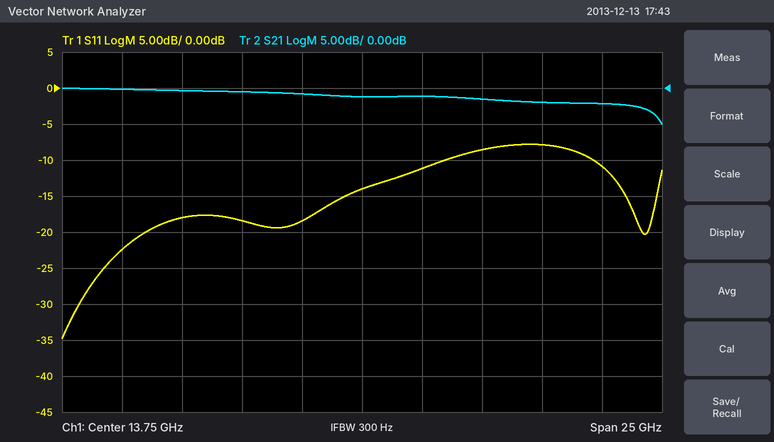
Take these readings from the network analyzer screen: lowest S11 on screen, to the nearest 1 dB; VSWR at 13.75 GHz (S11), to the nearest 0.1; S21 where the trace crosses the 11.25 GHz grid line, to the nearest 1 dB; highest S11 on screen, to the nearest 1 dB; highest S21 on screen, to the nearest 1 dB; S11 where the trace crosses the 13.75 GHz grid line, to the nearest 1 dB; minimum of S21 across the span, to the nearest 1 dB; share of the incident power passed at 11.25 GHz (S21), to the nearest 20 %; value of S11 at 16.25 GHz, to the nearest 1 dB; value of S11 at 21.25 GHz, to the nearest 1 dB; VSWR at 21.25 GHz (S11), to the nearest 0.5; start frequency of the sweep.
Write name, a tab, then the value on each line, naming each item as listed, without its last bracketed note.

lowest S11 on screen, to the nearest 1 dB	-35 dB
VSWR at 13.75 GHz (S11), to the nearest 0.1	1.5
S21 where the trace crosses the 11.25 GHz grid line, to the nearest 1 dB	-1 dB
highest S11 on screen, to the nearest 1 dB	-8 dB
highest S21 on screen, to the nearest 1 dB	0 dB
S11 where the trace crosses the 13.75 GHz grid line, to the nearest 1 dB	-14 dB
minimum of S21 across the span, to the nearest 1 dB	-5 dB
share of the incident power passed at 11.25 GHz (S21), to the nearest 20 %	80 %
value of S11 at 16.25 GHz, to the nearest 1 dB	-11 dB
value of S11 at 21.25 GHz, to the nearest 1 dB	-8 dB
VSWR at 21.25 GHz (S11), to the nearest 0.5	2.5
start frequency of the sweep	1.25 GHz
